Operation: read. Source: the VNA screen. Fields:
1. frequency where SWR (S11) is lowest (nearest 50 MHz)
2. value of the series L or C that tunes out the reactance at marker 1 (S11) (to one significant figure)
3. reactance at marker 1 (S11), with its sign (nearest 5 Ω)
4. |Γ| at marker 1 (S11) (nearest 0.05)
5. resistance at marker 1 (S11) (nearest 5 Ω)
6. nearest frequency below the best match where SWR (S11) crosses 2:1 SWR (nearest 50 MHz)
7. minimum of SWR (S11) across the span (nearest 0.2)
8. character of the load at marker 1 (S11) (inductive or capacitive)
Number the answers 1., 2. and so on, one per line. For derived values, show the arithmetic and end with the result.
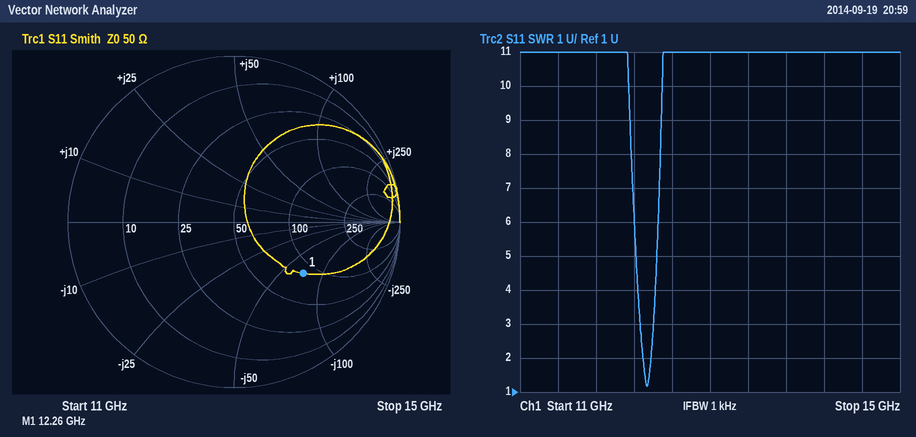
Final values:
1. 12.35 GHz
2. L = 70 Ω/(2π × 12.26 GHz) ≈ 909 pH, so 900 pH to one significant figure
3. -70 Ω
4. 0.50
5. 85 Ω
6. 12.30 GHz
7. 1.2
8. capacitive
